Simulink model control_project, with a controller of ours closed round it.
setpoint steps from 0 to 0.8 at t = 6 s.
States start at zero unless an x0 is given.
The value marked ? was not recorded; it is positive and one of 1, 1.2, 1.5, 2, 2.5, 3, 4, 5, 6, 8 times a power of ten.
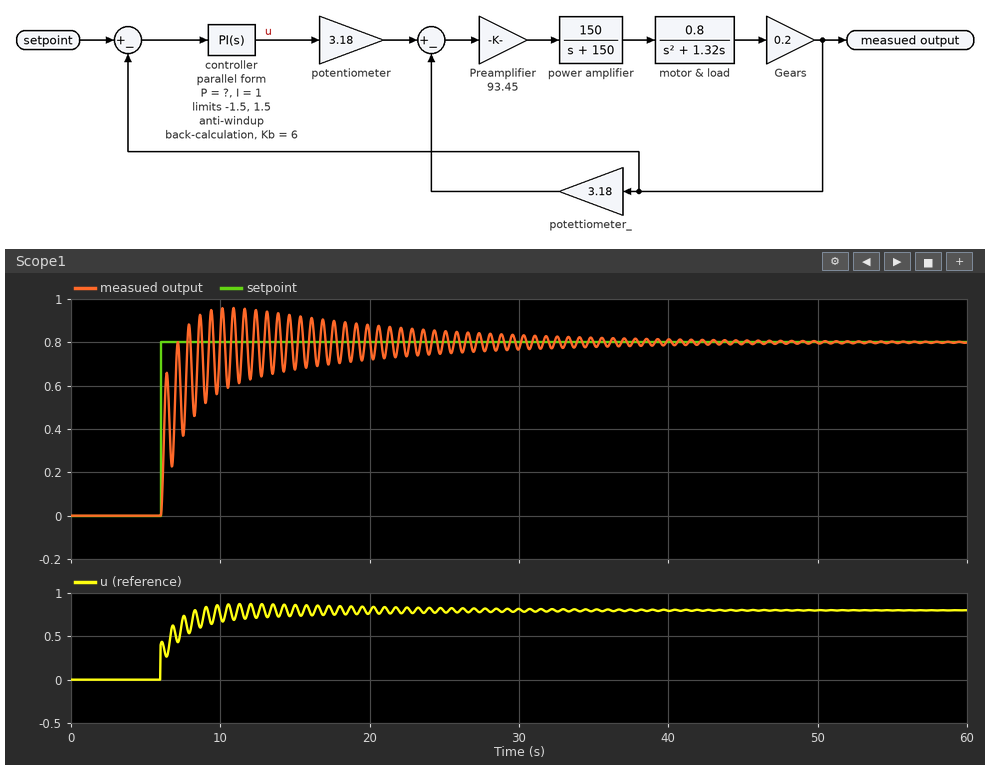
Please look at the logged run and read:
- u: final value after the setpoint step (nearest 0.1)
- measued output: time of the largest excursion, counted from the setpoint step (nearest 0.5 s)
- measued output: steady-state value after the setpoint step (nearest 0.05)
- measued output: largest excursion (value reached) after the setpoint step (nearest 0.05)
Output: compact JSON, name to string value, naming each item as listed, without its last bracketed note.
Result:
{"u: final value after the setpoint step": "0.8", "measued output: time of the largest excursion, counted from the setpoint step": "5.0 s", "measued output: steady-state value after the setpoint step": "0.80", "measued output: largest excursion (value reached) after the setpoint step": "0.95"}
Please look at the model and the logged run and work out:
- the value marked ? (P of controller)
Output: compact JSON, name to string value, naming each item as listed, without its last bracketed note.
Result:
{"the value marked ?": "0.5"}
